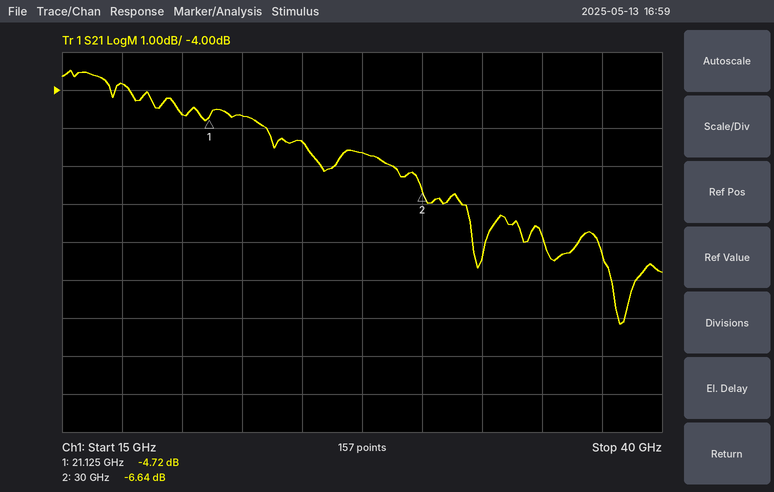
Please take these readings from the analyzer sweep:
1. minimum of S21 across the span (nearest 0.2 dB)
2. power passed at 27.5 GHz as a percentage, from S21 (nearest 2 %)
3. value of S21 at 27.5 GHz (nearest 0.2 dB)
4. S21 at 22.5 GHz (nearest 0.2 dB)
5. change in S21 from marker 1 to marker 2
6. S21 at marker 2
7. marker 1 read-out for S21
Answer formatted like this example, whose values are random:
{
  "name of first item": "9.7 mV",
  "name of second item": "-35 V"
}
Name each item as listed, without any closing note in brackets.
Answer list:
{
  "minimum of S21 across the span": "-10.2 dB",
  "power passed at 27.5 GHz as a percentage, from S21": "28 %",
  "value of S21 at 27.5 GHz": "-5.6 dB",
  "S21 at 22.5 GHz": "-4.6 dB",
  "change in S21 from marker 1 to marker 2": "-1.92 dB",
  "S21 at marker 2": "-6.64 dB",
  "marker 1 read-out for S21": "-4.72 dB"
}
